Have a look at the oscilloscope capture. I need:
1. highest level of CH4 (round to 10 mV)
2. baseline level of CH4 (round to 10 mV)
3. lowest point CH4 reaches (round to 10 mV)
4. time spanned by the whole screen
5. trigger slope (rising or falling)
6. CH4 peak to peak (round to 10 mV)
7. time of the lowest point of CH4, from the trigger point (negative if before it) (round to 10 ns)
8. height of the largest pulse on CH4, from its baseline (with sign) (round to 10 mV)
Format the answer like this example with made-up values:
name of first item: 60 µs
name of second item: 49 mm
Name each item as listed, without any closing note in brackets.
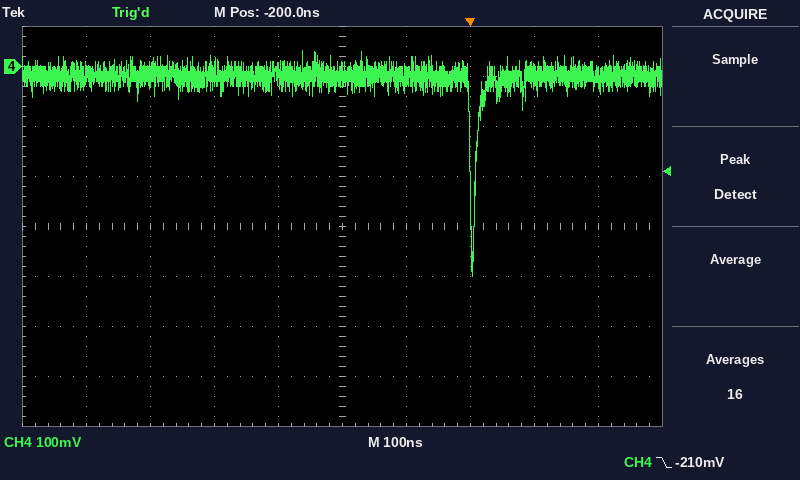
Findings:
highest level of CH4: 30 mV
baseline level of CH4: -20 mV
lowest point CH4 reaches: -420 mV
time spanned by the whole screen: 1 µs
trigger slope: falling
CH4 peak to peak: 450 mV
time of the lowest point of CH4, from the trigger point (negative if before it): 0 ns
height of the largest pulse on CH4, from its baseline (with sign): -400 mV
